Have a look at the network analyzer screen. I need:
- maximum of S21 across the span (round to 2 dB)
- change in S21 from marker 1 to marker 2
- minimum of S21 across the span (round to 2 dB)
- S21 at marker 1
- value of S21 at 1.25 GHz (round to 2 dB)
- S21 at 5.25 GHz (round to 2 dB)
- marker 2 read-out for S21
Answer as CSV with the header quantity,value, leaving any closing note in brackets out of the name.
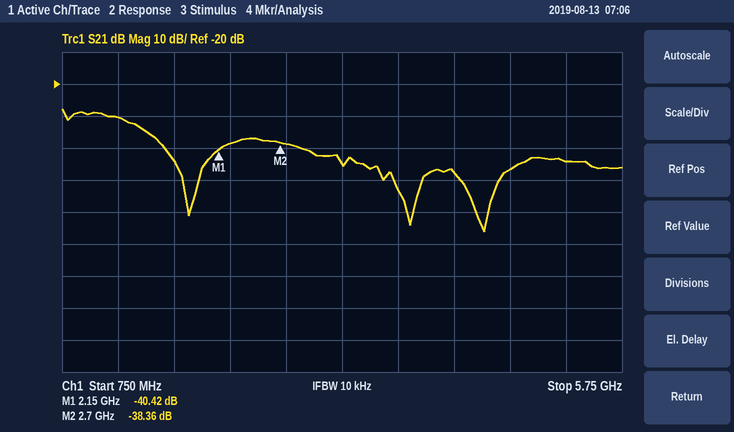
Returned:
quantity,value
maximum of S21 across the span,-28 dB
change in S21 from marker 1 to marker 2,2.06 dB
minimum of S21 across the span,-66 dB
S21 at marker 1,-40.42 dB
value of S21 at 1.25 GHz,-30 dB
S21 at 5.25 GHz,-44 dB
marker 2 read-out for S21,-38.36 dB
